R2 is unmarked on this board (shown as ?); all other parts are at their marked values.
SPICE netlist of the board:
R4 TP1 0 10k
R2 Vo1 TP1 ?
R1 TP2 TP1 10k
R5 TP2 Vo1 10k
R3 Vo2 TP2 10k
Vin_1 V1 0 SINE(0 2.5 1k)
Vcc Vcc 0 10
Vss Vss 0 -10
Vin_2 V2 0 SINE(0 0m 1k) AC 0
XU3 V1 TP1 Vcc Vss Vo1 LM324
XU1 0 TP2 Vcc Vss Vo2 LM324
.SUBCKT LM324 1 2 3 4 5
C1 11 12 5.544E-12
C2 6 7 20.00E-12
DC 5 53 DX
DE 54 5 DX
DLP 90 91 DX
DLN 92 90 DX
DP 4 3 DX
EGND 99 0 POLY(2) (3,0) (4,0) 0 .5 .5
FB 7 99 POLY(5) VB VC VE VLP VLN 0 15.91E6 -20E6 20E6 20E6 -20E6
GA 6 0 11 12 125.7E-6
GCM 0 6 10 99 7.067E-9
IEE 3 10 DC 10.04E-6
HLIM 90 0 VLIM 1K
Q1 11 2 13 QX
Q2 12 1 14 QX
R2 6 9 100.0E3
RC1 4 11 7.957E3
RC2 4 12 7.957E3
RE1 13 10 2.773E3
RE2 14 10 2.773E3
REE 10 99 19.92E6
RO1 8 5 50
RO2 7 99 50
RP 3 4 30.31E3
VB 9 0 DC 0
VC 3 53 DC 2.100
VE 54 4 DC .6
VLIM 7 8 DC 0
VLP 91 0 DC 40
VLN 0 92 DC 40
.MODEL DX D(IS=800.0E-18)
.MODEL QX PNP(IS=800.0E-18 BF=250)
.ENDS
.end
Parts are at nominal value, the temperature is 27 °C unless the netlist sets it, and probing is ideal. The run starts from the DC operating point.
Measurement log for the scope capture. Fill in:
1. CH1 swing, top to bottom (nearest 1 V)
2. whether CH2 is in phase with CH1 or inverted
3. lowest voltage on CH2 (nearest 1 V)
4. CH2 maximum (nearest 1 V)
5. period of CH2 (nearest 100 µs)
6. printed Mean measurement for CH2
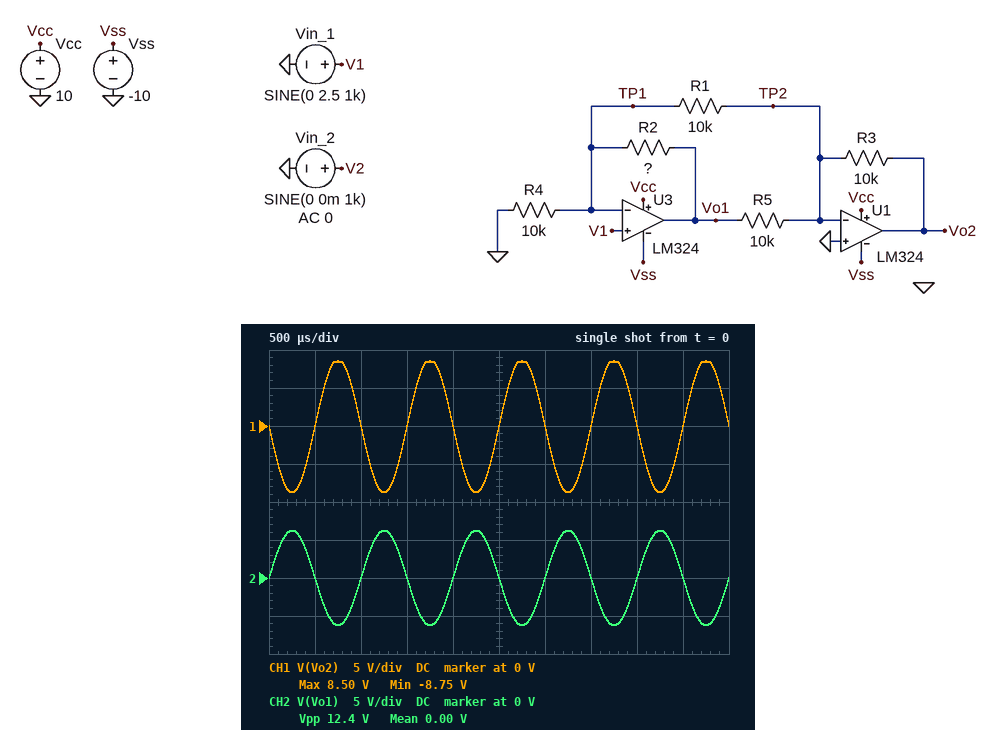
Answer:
17 V
inverted
-6 V
6 V
1.0 ms
0.00 V
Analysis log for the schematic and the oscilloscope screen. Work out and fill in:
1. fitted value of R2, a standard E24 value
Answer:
7.5 kΩ
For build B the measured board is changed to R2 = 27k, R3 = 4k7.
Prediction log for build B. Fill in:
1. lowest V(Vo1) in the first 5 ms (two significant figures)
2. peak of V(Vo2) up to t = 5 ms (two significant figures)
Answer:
-10 V
5.4 V
